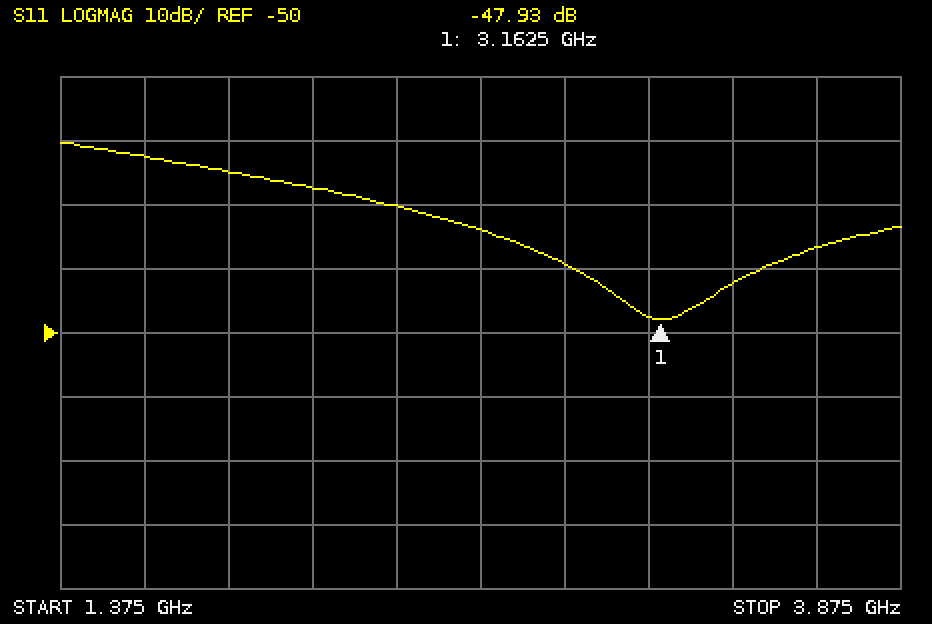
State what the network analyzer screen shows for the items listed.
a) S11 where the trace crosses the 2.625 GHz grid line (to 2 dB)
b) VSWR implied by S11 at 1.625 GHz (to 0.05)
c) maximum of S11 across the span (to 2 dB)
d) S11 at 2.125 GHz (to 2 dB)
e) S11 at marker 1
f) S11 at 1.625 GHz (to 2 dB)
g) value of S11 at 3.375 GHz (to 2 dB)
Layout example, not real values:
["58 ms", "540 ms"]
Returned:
["-34 dB", "1.15", "-20 dB", "-28 dB", "-47.93 dB", "-22 dB", "-42 dB"]
